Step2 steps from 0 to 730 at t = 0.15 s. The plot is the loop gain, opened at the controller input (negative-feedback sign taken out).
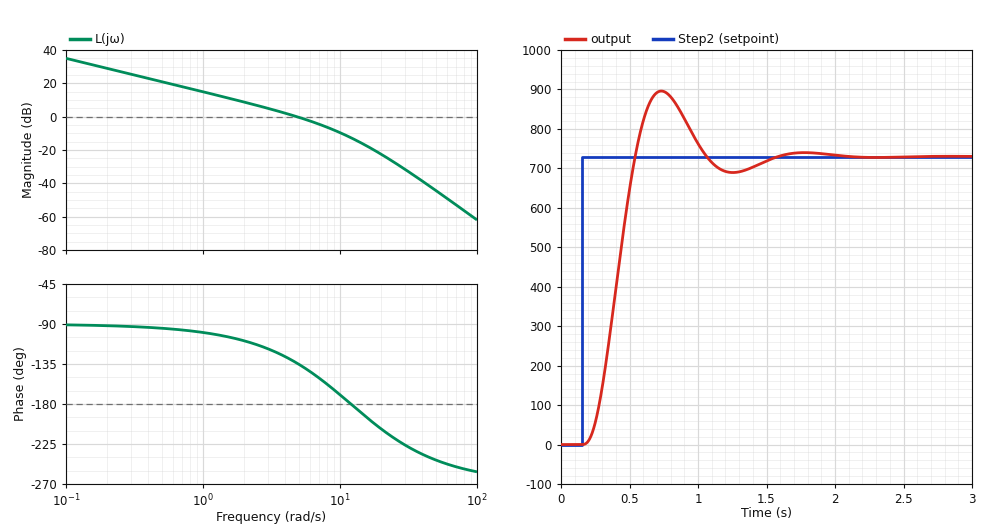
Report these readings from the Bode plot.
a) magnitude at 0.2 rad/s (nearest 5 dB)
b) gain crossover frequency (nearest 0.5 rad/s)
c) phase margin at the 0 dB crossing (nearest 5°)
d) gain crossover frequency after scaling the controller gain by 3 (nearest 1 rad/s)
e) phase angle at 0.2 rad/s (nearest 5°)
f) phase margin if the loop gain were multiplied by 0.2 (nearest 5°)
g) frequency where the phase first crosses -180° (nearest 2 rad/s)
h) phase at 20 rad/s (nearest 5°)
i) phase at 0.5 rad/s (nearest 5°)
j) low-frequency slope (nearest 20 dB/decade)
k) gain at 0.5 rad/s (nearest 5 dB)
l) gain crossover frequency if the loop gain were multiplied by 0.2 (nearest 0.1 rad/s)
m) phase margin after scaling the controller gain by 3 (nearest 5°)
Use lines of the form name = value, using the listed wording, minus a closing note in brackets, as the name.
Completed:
magnitude at 0.2 rad/s = 30 dB
gain crossover frequency = 5.0 rad/s
phase margin at the 0 dB crossing = 45°
gain crossover frequency after scaling the controller gain by 3 = 10 rad/s
phase angle at 0.2 rad/s = -90°
phase margin if the loop gain were multiplied by 0.2 = 80°
frequency where the phase first crosses -180° = 12 rad/s
phase at 20 rad/s = -210°
phase at 0.5 rad/s = -95°
low-frequency slope = -20 dB/decade
gain at 0.5 rad/s = 20 dB
gain crossover frequency if the loop gain were multiplied by 0.2 = 1.1 rad/s
phase margin after scaling the controller gain by 3 = 10°
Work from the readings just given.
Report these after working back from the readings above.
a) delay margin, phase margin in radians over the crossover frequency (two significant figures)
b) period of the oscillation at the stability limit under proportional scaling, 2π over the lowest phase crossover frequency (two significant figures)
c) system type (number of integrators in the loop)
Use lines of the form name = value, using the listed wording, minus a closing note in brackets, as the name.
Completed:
delay margin, phase margin in radians over the crossover frequency = 0.16 s
period of the oscillation at the stability limit under proportional scaling, 2π over the lowest phase crossover frequency = 0.52 s
system type = 1
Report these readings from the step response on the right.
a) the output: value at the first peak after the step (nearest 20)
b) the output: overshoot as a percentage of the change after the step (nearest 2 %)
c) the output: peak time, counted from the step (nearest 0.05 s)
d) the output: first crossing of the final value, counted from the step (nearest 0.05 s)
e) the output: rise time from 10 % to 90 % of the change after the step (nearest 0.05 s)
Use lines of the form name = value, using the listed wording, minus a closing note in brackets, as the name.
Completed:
the output: value at the first peak after the step = 900
the output: overshoot as a percentage of the change after the step = 22 %
the output: peak time, counted from the step = 0.60 s
the output: first crossing of the final value, counted from the step = 0.40 s
the output: rise time from 10 % to 90 % of the change after the step = 0.25 s
